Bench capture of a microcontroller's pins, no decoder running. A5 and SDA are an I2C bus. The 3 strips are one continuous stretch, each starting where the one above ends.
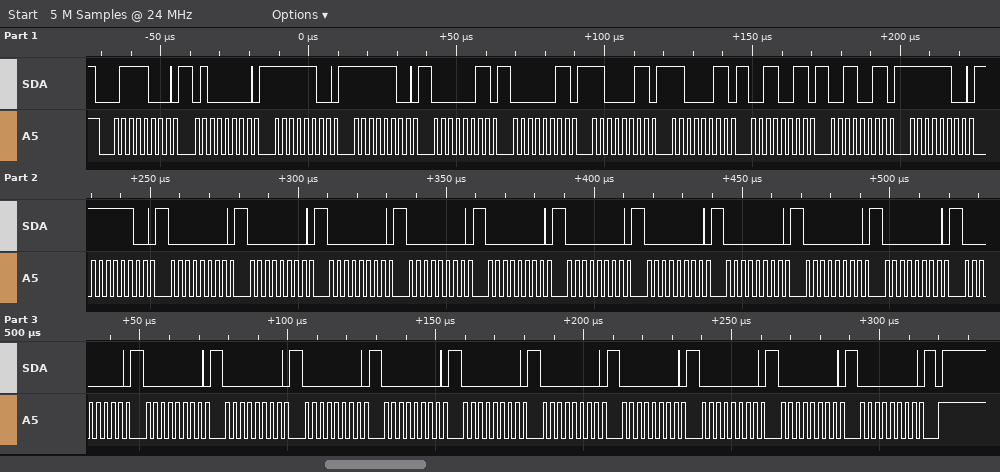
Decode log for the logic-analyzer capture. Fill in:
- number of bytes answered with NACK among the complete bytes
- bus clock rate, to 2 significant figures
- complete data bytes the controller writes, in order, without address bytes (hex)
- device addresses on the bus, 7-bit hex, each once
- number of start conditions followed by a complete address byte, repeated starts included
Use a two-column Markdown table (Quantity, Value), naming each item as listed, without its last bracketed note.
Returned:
| Quantity | Value |
|---|---|
| number of bytes answered with NACK among the complete bytes | 0 |
| bus clock rate, to 2 significant figures | 400 kHz |
| complete data bytes the controller writes, in order, without address bytes | 40 FC FC 03 03 C3 C3 33 33 FC FC 00 00 00 00 00 00 00 00 00 00 00 00 00 00 00 00 00 00 00 00 00 |
| device addresses on the bus, 7-bit hex, each once | 0x3C |
| number of start conditions followed by a complete address byte, repeated starts included | 1 |
